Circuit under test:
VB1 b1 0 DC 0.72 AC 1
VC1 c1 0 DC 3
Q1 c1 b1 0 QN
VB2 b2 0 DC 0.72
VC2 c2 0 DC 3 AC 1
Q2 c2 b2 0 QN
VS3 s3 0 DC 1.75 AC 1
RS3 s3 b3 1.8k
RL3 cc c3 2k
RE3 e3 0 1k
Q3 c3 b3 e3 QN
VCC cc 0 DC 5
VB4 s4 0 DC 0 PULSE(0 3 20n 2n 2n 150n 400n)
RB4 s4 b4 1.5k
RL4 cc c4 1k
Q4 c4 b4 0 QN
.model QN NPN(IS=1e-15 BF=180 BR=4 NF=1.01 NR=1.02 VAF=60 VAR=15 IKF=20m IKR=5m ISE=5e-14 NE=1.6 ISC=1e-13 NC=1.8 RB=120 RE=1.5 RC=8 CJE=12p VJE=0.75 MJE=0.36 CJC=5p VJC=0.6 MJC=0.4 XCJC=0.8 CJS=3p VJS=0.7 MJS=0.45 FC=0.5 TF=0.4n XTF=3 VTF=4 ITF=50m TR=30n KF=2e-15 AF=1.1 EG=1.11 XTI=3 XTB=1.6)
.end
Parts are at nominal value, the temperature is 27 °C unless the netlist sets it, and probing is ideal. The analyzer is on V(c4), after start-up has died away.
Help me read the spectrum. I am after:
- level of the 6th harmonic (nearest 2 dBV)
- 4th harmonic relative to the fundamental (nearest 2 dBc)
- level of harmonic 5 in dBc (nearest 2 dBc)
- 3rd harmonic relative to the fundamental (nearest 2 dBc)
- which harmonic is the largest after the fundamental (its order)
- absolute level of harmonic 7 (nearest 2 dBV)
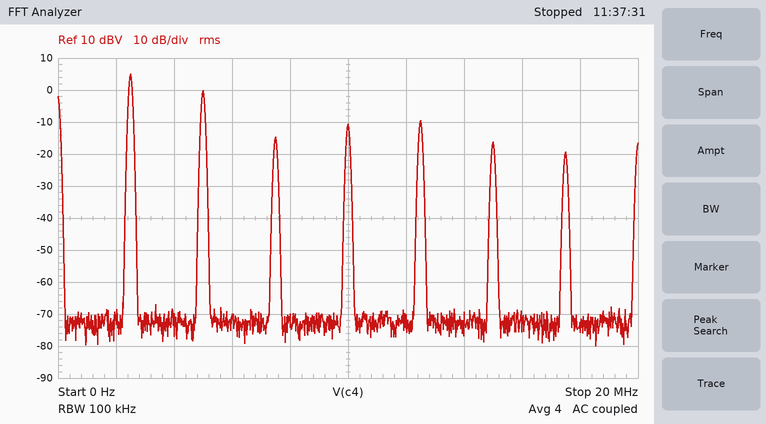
-16 dBV
-16 dBc
-14 dBc
-20 dBc
2
-20 dBV
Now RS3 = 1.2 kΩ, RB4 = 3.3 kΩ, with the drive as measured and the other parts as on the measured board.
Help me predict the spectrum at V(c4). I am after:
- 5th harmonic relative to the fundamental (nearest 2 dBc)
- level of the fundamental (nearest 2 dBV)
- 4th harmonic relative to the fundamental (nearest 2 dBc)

-20 dBc
4 dBV
-18 dBc
